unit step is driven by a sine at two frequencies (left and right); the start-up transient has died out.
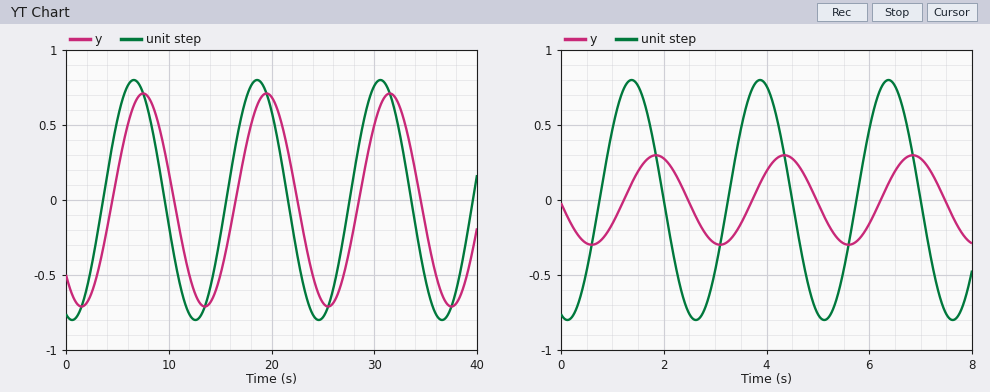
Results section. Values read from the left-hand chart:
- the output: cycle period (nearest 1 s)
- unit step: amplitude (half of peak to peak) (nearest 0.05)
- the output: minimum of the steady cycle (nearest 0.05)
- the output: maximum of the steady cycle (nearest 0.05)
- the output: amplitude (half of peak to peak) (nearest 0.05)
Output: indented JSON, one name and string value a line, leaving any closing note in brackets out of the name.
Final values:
{
  "the output: cycle period": "12 s",
  "unit step: amplitude (half of peak to peak)": "0.80",
  "the output: minimum of the steady cycle": "-0.70",
  "the output: maximum of the steady cycle": "0.70",
  "the output: amplitude (half of peak to peak)": "0.70"
}
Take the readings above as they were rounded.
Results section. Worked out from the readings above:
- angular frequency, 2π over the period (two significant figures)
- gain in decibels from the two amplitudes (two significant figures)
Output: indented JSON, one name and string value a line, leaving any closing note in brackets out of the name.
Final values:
{
  "angular frequency, 2π over the period": "0.52 rad/s",
  "gain in decibels from the two amplitudes": "-1.2 dB"
}
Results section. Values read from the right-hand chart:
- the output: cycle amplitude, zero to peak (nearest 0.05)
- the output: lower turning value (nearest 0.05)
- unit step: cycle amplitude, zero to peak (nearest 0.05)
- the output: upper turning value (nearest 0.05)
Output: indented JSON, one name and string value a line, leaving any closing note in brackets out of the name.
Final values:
{
  "the output: cycle amplitude, zero to peak": "0.30",
  "the output: lower turning value": "-0.30",
  "unit step: cycle amplitude, zero to peak": "0.80",
  "the output: upper turning value": "0.30"
}
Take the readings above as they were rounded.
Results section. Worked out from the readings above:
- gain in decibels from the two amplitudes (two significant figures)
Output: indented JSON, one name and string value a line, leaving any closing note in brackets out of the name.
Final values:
{
  "gain in decibels from the two amplitudes": "-8.5 dB"
}
